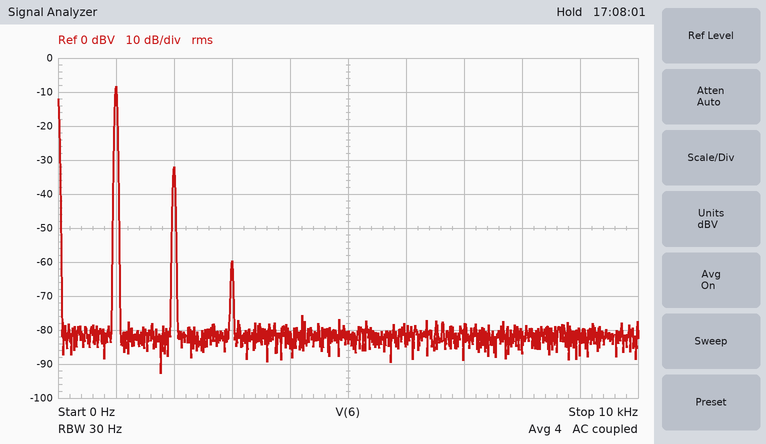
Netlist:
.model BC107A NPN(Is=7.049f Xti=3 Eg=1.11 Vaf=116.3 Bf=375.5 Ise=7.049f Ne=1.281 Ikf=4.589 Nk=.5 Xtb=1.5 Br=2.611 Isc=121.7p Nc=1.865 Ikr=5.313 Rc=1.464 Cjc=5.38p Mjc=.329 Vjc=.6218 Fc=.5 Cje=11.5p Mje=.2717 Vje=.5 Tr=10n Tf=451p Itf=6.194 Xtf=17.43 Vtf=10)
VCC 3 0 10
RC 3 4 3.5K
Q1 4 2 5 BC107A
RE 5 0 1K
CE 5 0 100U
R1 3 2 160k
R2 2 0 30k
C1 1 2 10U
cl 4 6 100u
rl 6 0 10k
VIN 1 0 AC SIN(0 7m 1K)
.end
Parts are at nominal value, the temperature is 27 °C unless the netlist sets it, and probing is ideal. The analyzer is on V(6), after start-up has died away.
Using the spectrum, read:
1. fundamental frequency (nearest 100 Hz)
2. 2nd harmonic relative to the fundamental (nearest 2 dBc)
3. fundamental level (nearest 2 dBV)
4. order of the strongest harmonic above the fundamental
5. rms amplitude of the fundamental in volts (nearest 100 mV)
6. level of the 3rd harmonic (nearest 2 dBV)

1.0 kHz
-24 dBc
-8 dBV
2
400 mV
-60 dBV
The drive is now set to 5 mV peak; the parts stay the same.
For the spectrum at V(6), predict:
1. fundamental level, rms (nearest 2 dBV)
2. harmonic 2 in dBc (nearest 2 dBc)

-12 dBV
-26 dBc
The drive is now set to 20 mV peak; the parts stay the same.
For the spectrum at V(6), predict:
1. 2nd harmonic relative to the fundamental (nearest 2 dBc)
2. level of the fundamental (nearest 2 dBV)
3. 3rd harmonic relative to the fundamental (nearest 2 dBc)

-14 dBc
0 dBV
-34 dBc
